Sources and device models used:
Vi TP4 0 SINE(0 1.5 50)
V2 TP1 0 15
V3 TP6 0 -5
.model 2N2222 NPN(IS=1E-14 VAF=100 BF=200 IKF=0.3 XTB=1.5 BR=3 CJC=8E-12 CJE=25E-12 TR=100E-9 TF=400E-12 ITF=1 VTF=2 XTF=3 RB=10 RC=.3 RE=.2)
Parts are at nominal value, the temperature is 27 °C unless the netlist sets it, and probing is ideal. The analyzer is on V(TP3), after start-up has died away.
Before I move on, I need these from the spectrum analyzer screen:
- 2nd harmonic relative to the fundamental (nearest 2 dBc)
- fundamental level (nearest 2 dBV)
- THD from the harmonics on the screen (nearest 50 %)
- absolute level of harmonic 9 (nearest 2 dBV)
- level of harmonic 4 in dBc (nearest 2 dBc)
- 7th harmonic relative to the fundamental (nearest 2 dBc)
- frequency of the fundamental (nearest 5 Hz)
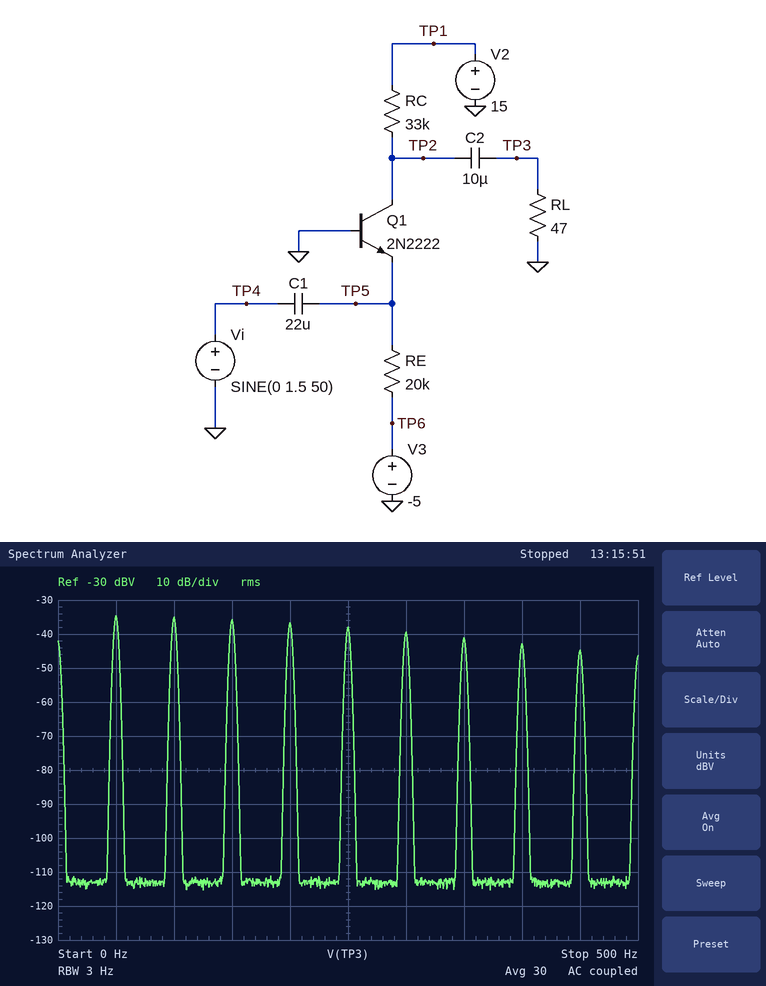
0 dBc
-34 dBV
200 %
-44 dBV
-2 dBc
-6 dBc
50 Hz
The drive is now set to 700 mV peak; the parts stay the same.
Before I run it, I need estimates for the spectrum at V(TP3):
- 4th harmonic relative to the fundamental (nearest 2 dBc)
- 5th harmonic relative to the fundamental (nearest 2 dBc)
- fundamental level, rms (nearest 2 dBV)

-4 dBc
-6 dBc
-36 dBV
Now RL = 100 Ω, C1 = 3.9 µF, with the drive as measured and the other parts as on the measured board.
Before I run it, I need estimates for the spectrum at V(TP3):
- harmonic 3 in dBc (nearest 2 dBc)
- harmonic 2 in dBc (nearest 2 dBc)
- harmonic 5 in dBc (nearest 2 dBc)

-4 dBc
-2 dBc
-12 dBc
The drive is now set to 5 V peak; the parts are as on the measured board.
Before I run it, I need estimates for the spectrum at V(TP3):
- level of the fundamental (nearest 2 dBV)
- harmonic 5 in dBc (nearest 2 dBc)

-30 dBV
-2 dBc
